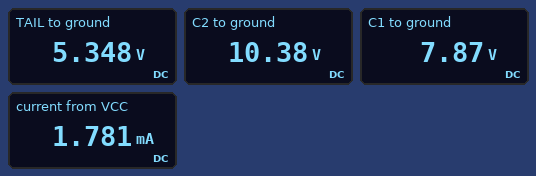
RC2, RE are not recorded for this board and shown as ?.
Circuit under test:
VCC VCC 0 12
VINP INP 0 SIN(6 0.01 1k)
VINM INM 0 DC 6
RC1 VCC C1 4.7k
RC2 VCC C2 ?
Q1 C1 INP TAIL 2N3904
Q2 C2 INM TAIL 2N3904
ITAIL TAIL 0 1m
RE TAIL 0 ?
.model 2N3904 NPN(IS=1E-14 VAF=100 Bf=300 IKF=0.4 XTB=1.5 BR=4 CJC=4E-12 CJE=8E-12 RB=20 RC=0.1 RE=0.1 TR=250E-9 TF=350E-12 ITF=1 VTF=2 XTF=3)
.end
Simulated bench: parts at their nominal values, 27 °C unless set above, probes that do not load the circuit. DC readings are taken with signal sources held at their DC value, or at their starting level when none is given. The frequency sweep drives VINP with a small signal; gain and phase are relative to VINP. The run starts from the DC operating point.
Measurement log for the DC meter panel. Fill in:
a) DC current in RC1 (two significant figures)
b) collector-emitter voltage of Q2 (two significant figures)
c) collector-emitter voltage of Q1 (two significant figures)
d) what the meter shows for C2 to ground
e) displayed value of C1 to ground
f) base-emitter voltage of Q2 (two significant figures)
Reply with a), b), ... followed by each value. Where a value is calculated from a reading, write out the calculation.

a) (12 V - 7.87 V) / 4.7 kΩ = 880 µA
b) 10.38 V - 5.348 V = 5.0 V
c) 7.87 V - 5.348 V = 2.5 V
d) 10.38 V
e) 7.87 V
f) 6 V - 5.348 V = 650 mV
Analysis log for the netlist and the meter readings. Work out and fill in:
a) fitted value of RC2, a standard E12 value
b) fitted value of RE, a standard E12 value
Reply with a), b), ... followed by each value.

a) 1.8 kΩ
b) 6.8 kΩ
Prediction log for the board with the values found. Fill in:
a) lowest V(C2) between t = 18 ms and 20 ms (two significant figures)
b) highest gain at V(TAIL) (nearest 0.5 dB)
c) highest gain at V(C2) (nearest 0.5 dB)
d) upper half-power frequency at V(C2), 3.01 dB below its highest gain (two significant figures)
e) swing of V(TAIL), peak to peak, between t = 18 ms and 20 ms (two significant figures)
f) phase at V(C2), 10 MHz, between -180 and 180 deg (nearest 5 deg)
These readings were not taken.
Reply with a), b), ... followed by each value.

a) 10 V
b) -6.0 dB
c) 29.5 dB
d) 18 MHz
e) 9.7 mV
f) -25 deg
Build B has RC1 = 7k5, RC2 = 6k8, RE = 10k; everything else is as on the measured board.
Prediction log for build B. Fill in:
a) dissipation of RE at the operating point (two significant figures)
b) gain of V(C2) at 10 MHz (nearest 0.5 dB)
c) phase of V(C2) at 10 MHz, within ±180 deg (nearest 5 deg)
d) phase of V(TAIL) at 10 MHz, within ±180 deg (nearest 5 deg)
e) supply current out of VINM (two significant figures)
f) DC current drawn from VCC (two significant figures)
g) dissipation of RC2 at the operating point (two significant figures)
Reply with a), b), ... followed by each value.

a) 2.9 mW
b) 32.0 dB
c) -65 deg
d) 0 deg
e) 2.5 µA
f) 1.5 mA
g) 4.0 mW
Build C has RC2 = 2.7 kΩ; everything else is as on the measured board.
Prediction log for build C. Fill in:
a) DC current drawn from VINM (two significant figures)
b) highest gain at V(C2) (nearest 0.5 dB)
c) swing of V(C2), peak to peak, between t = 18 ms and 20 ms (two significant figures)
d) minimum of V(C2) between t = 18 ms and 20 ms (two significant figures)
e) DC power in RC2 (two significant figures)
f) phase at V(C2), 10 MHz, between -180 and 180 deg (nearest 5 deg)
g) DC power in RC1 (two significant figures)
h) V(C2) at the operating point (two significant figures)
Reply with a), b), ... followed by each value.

a) 2.9 µA
b) 33.0 dB
c) 880 mV
d) 9.1 V
e) 2.2 mW
f) -35 deg
g) 3.7 mW
h) 9.6 V
